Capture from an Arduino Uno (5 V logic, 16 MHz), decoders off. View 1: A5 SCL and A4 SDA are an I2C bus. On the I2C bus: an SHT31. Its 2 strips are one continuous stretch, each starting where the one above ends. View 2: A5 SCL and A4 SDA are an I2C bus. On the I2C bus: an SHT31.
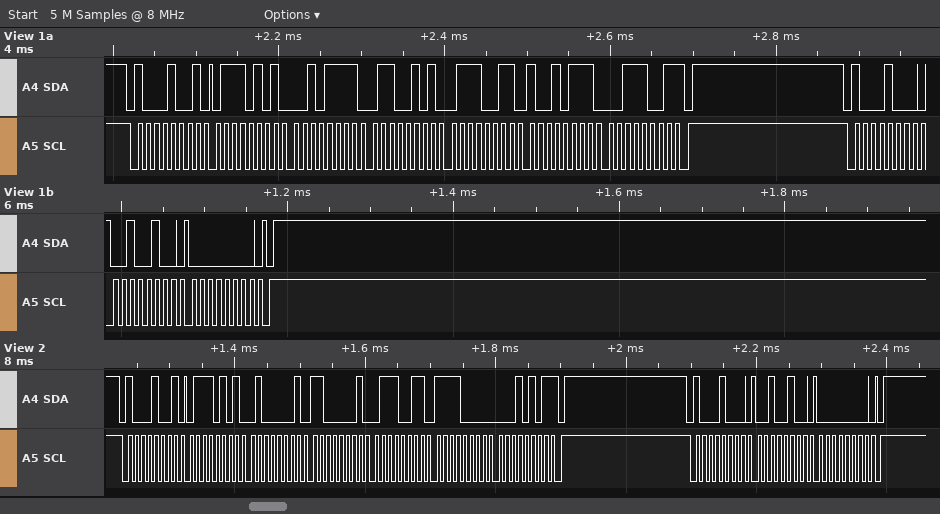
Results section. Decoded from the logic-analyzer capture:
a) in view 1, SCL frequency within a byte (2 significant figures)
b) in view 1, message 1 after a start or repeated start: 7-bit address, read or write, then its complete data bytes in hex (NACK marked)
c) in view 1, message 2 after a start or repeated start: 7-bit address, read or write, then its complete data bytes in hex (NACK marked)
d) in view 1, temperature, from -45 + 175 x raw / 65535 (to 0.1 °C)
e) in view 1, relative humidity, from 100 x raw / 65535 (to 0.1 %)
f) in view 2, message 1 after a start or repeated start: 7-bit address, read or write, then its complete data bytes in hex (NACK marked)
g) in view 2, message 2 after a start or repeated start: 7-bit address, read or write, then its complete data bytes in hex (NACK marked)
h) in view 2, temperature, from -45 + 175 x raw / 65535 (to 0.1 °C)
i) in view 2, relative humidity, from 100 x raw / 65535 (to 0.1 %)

100 kHz
0x44 read: 75 2F 65 73 97 39 NACK
0x44 write: 24 00
35.1 °C
45.2 %
0x44 read: 75 41 C1 73 F0 15 NACK
0x44 write: 24 00
35.2 °C
45.3 %
